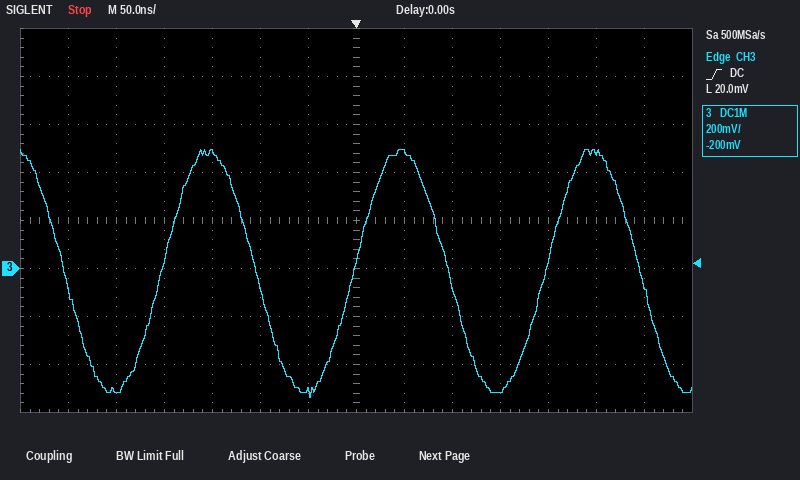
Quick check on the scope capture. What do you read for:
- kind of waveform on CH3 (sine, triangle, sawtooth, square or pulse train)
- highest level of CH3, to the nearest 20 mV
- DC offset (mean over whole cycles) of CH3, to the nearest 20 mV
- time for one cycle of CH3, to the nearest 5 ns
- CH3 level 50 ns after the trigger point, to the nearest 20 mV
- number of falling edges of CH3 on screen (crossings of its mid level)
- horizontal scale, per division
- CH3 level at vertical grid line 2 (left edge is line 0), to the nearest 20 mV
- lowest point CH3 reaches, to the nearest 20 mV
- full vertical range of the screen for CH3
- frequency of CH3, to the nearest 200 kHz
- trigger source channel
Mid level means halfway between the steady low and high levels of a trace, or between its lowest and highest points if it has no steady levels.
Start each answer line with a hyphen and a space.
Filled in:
- sine
- 500 mV
- -20 mV
- 200 ns
- 480 mV
- 4
- 50 ns
- -520 mV
- -540 mV
- 1.6 V
- 5.0 MHz
- CH3
